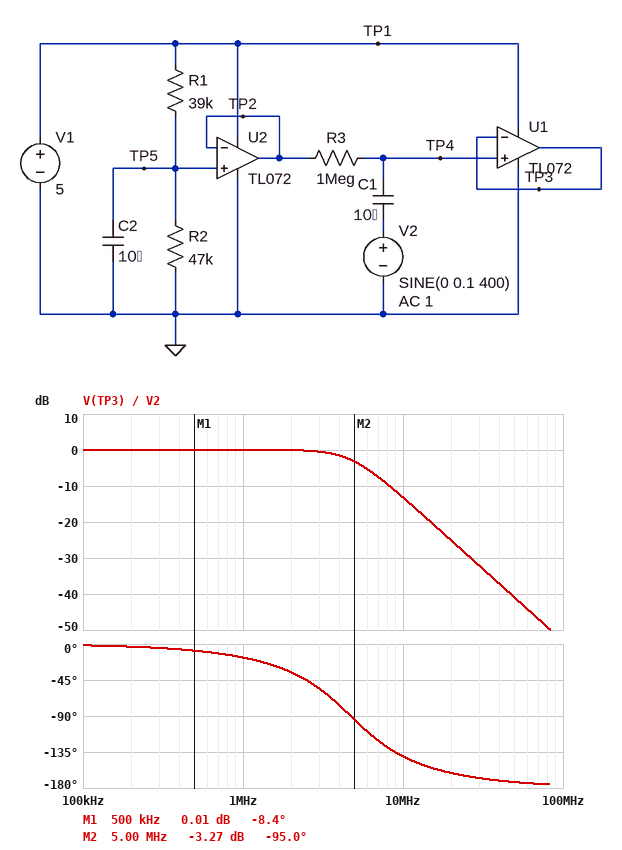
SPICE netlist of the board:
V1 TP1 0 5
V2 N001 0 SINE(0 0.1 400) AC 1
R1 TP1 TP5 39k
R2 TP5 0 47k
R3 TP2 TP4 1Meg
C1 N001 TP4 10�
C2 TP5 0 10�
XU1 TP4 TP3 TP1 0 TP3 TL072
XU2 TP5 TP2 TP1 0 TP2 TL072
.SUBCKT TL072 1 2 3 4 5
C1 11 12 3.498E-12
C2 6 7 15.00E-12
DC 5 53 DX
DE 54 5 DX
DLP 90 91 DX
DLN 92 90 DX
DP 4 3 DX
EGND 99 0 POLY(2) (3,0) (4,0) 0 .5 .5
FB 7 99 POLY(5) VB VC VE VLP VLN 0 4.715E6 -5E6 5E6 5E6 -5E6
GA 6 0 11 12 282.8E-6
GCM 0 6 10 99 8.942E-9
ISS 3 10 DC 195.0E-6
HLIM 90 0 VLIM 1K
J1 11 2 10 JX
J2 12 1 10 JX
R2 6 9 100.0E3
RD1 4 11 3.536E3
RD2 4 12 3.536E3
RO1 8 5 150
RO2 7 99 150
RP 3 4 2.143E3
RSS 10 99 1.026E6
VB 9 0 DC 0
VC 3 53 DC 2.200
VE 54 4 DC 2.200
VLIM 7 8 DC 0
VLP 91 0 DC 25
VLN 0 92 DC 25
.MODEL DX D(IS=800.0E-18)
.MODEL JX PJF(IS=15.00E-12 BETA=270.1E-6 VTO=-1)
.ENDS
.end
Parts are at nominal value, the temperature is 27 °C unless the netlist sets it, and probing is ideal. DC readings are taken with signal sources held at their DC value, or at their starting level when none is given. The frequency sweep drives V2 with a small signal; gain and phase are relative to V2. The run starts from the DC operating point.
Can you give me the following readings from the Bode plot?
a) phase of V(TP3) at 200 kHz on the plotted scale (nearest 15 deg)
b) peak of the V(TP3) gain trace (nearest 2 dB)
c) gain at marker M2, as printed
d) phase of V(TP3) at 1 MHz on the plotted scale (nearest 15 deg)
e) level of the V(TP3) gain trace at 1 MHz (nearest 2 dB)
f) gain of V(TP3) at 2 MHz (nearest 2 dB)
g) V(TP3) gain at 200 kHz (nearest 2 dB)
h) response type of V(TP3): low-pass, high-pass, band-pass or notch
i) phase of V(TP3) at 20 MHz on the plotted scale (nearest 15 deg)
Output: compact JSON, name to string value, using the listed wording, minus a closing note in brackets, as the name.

{"phase of V(TP3) at 200 kHz on the plotted scale": "0 deg", "peak of the V(TP3) gain trace": "0 dB", "gain at marker M2, as printed": "-3.27 dB", "phase of V(TP3) at 1 MHz on the plotted scale": "-15 deg", "level of the V(TP3) gain trace at 1 MHz": "0 dB", "gain of V(TP3) at 2 MHz": "0 dB", "V(TP3) gain at 200 kHz": "0 dB", "response type of V(TP3): low-pass, high-pass, band-pass or notch": "low-pass", "phase of V(TP3) at 20 MHz on the plotted scale": "-165 deg"}
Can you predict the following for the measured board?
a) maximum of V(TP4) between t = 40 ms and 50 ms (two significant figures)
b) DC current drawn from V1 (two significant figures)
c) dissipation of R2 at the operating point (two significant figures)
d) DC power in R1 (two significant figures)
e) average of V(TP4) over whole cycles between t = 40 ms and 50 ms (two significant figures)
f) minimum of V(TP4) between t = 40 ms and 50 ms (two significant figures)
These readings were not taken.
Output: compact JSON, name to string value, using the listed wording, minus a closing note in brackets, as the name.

{"maximum of V(TP4) between t = 40 ms and 50 ms": "2.8 V", "DC current drawn from V1": "5.1 mA", "dissipation of R2 at the operating point": "160 µW", "DC power in R1": "130 µW", "average of V(TP4) over whole cycles between t = 40 ms and 50 ms": "2.7 V", "minimum of V(TP4) between t = 40 ms and 50 ms": "2.6 V"}
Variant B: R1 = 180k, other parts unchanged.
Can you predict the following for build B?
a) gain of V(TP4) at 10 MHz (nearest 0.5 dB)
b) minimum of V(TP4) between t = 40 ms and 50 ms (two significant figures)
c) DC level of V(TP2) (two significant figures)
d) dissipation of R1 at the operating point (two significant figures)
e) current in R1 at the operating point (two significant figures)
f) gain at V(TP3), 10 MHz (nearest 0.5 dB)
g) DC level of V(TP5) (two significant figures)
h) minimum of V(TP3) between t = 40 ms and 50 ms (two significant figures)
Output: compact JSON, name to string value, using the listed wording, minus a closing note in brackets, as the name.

{"gain of V(TP4) at 10 MHz": "0 dB", "minimum of V(TP4) between t = 40 ms and 50 ms": "1.4 V", "DC level of V(TP2)": "1.5 V", "dissipation of R1 at the operating point": "87 µW", "current in R1 at the operating point": "22 µA", "gain at V(TP3), 10 MHz": "-50.5 dB", "DC level of V(TP5)": "1.0 V", "minimum of V(TP3) between t = 40 ms and 50 ms": "1.6 V"}
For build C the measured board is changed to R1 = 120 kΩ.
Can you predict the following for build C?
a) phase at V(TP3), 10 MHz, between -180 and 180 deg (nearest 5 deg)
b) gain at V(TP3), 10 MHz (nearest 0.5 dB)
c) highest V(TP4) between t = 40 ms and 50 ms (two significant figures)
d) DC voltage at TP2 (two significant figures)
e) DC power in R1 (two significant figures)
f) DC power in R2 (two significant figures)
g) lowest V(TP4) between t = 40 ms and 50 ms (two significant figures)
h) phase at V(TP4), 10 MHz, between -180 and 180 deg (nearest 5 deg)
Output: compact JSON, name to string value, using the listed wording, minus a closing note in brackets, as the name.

{"phase at V(TP3), 10 MHz, between -180 and 180 deg": "-145 deg", "gain at V(TP3), 10 MHz": "-48.0 dB", "highest V(TP4) between t = 40 ms and 50 ms": "1.7 V", "DC voltage at TP2": "1.6 V", "DC power in R1": "110 µW", "DC power in R2": "42 µW", "lowest V(TP4) between t = 40 ms and 50 ms": "1.5 V", "phase at V(TP4), 10 MHz, between -180 and 180 deg": "0 deg"}
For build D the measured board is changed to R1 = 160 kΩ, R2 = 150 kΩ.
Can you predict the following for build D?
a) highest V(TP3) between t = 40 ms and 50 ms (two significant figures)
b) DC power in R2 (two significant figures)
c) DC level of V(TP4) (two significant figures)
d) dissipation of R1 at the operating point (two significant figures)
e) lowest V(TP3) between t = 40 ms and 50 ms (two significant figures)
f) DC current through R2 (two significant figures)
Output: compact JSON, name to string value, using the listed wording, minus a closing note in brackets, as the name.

{"highest V(TP3) between t = 40 ms and 50 ms": "2.5 V", "DC power in R2": "39 µW", "DC level of V(TP4)": "2.4 V", "dissipation of R1 at the operating point": "42 µW", "lowest V(TP3) between t = 40 ms and 50 ms": "2.3 V", "DC current through R2": "16 µA"}
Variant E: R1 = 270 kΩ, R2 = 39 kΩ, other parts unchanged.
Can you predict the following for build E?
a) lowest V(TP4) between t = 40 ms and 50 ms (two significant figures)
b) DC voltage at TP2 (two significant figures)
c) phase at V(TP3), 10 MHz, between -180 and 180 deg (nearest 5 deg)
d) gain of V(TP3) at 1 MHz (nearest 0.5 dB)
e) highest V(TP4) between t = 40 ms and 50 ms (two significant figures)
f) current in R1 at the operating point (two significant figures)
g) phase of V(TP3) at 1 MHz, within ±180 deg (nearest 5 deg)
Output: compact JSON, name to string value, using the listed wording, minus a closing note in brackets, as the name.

{"lowest V(TP4) between t = 40 ms and 50 ms": "1.4 V", "DC voltage at TP2": "1.5 V", "phase at V(TP3), 10 MHz, between -180 and 180 deg": "-145 deg", "gain of V(TP3) at 1 MHz": "-26.0 dB", "highest V(TP4) between t = 40 ms and 50 ms": "1.6 V", "current in R1 at the operating point": "16 µA", "phase of V(TP3) at 1 MHz, within ±180 deg": "-90 deg"}
